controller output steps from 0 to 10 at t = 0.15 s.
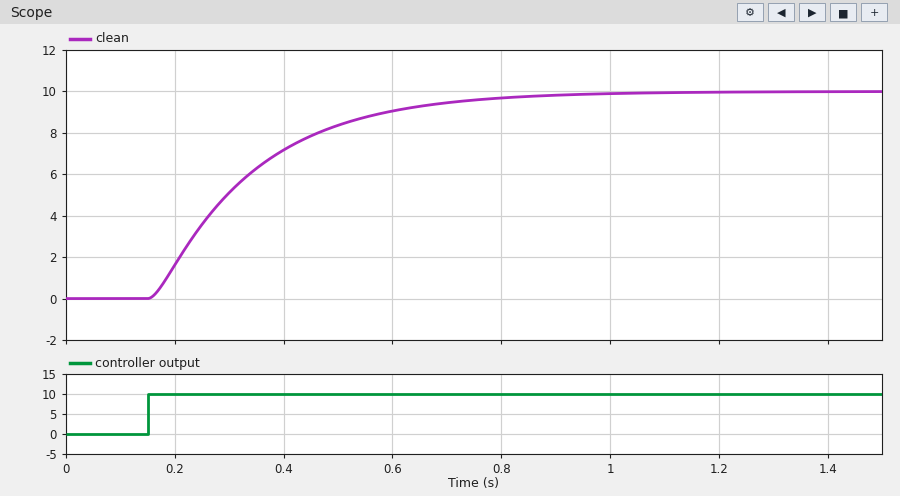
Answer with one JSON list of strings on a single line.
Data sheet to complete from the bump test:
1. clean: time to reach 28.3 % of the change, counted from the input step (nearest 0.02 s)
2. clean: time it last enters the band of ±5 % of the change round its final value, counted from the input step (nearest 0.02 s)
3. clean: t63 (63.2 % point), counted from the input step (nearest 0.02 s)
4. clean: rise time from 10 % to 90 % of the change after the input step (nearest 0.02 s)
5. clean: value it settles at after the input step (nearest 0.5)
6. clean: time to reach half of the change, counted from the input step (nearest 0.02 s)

["0.08 s", "0.56 s", "0.20 s", "0.40 s", "10.0", "0.14 s"]
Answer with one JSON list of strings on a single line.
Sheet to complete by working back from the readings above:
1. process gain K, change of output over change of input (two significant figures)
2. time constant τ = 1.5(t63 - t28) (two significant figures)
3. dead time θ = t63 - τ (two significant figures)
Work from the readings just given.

["1.0", "0.18 s", "0.020 s"]
